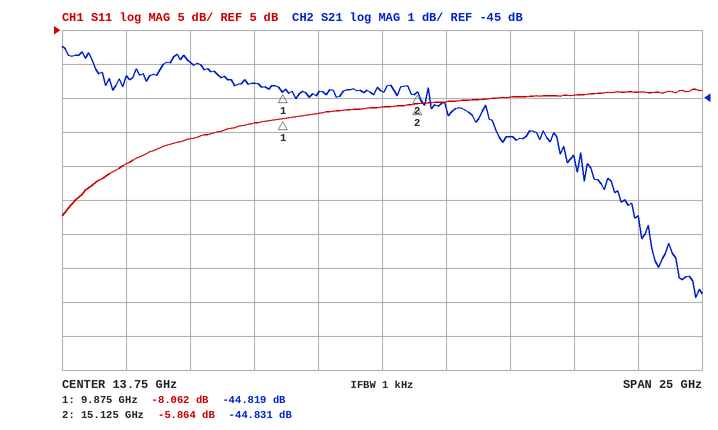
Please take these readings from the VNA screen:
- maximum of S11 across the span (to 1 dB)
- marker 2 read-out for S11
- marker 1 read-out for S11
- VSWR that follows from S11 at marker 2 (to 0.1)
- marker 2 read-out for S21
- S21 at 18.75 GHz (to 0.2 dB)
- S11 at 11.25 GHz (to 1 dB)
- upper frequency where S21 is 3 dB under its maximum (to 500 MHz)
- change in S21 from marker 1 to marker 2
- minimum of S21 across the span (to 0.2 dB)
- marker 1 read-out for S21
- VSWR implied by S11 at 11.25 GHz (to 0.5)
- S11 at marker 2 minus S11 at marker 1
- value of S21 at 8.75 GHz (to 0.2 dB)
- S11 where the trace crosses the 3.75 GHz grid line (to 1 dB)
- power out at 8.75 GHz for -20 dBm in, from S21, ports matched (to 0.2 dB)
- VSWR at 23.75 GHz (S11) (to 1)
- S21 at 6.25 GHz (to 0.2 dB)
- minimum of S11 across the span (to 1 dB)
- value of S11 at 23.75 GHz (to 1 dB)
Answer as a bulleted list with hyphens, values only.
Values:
- -4 dB
- -5.864 dB
- -8.062 dB
- 3.1
- -44.831 dB
- -46.2 dB
- -7 dB
- 20.5 GHz
- -0.012 dB
- -50.8 dB
- -44.819 dB
- 2.5
- 2.198 dB
- -44.6 dB
- -15 dB
- -64.6 dBm
- 4
- -44.0 dB
- -22 dB
- -4 dB
